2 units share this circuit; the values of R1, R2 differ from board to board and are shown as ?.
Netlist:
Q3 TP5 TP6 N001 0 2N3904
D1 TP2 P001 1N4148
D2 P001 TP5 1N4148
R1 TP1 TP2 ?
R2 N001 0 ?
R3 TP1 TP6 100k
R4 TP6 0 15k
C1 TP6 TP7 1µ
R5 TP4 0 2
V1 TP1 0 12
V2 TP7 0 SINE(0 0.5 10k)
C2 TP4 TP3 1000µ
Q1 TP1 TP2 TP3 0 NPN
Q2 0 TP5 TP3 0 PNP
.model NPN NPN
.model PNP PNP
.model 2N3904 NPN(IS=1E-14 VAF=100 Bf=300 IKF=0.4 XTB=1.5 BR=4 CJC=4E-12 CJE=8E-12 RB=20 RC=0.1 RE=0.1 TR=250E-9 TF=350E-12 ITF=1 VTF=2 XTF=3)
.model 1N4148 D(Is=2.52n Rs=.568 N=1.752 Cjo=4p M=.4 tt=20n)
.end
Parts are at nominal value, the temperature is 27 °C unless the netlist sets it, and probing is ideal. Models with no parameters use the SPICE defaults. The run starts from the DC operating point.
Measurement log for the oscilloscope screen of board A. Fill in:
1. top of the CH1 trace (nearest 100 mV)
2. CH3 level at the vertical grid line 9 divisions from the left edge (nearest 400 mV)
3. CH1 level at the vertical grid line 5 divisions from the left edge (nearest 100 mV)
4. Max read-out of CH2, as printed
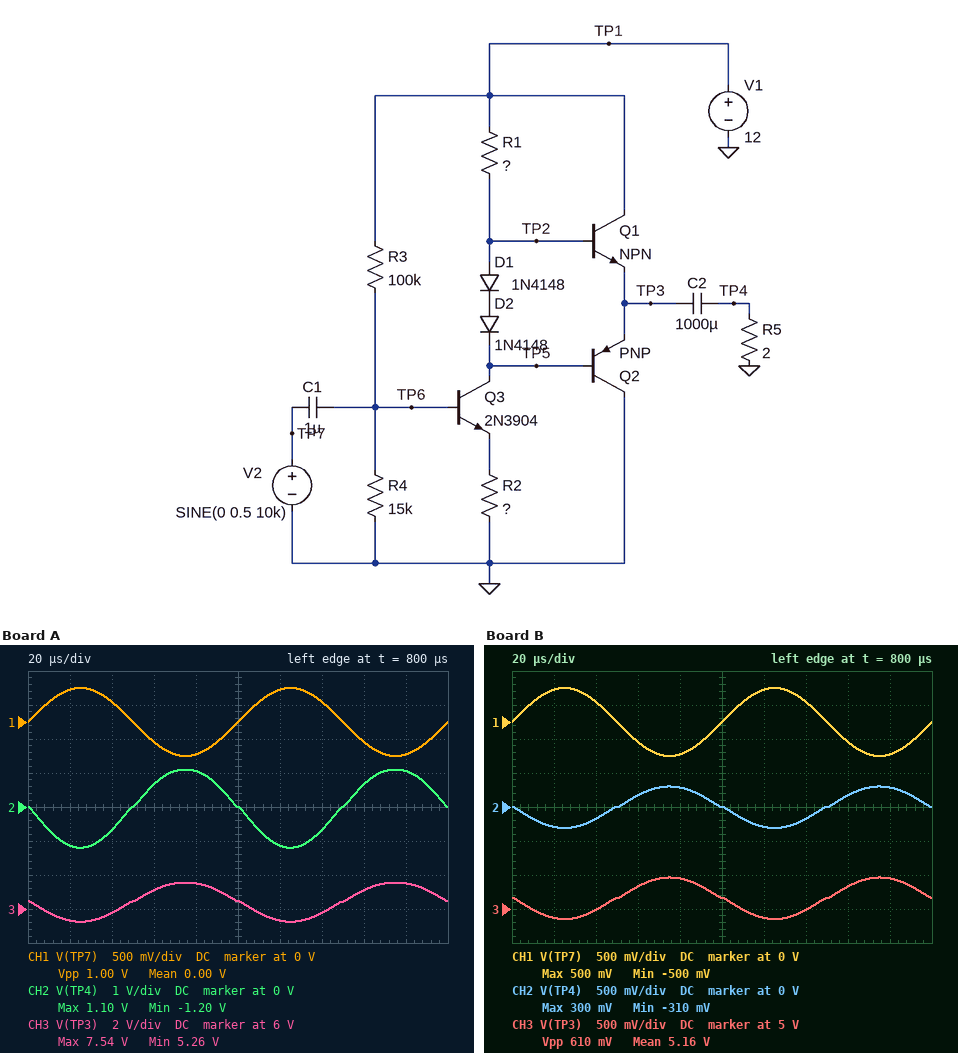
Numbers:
500 mV
7.6 V
0 V
1.10 V
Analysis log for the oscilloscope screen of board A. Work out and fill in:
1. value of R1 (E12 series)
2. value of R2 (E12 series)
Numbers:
560 Ω
56 Ω
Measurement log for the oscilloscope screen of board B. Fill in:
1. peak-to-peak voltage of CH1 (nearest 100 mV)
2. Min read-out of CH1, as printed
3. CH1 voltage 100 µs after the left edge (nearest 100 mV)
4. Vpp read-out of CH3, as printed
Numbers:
1.0 V
-500 mV
0 V
610 mV
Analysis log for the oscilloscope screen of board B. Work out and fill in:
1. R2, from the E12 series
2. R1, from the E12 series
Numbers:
270 Ω
2.2 kΩ
